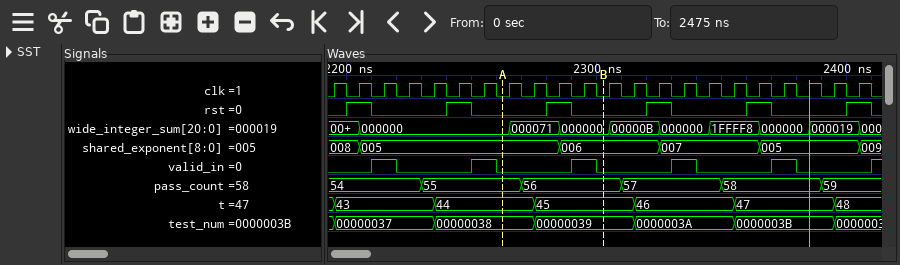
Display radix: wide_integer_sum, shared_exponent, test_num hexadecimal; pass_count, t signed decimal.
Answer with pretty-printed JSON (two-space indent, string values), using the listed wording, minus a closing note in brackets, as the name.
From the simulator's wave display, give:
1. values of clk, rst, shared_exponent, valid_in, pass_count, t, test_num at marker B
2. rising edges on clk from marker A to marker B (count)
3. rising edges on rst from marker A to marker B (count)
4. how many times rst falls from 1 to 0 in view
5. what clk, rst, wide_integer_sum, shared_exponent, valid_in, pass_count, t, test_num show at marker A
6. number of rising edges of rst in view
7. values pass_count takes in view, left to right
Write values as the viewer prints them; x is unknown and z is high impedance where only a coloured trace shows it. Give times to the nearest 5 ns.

{
  "values of clk, rst, shared_exponent, valid_in, pass_count, t, test_num at marker B": "clk=0, rst=0, shared_exponent=006, valid_in=0, pass_count=56, t=45, test_num=00000039",
  "rising edges on clk from marker A to marker B": "4",
  "rising edges on rst from marker A to marker B": "1",
  "how many times rst falls from 1 to 0 in view": "6",
  "what clk, rst, wide_integer_sum, shared_exponent, valid_in, pass_count, t, test_num show at marker A": "clk=0, rst=0, wide_integer_sum=000000, shared_exponent=005, valid_in=0, pass_count=55, t=44, test_num=00000038",
  "number of rising edges of rst in view": "6",
  "values pass_count takes in view, left to right": "54, 55, 56, 57, 58, 59"
}
